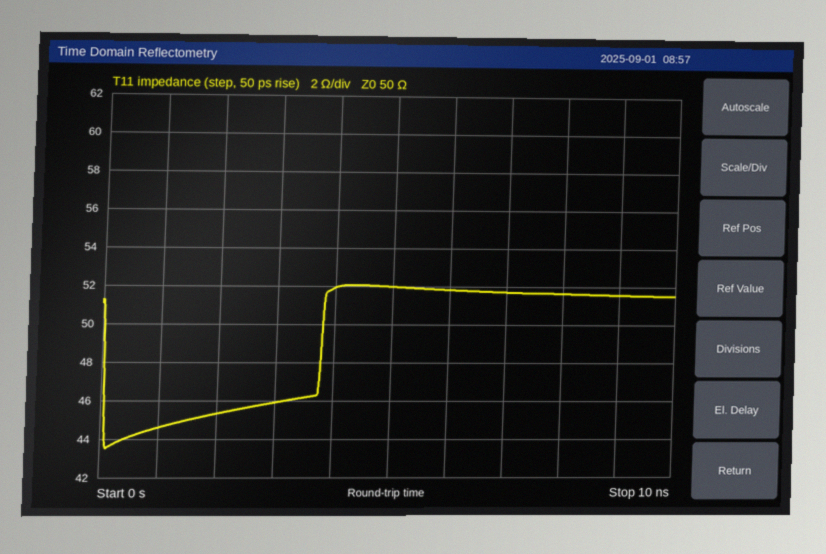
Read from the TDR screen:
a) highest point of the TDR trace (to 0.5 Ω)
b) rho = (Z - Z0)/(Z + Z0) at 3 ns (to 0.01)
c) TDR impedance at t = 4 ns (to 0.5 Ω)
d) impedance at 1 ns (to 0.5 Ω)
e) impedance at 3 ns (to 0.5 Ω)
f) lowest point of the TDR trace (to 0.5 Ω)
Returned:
52.0 Ω
-0.04
52.0 Ω
44.5 Ω
46.0 Ω
43.5 Ω
